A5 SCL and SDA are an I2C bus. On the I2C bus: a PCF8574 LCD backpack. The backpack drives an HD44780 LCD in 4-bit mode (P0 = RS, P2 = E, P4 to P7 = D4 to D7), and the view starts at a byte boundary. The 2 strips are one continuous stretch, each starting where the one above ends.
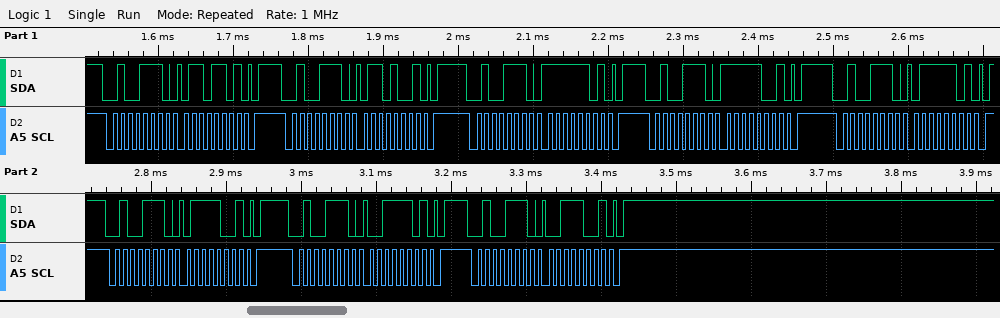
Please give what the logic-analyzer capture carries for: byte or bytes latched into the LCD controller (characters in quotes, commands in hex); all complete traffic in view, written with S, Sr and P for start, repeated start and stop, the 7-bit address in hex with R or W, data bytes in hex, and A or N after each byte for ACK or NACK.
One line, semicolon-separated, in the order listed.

'o' 's'; S 27W A 6D A P S 27W A 69 A P S 27W A FD A P S 27W A F9 A P S 27W A 7D A P S 27W A 79 A P S 27W A 3D A P S 27W A 39 A P
